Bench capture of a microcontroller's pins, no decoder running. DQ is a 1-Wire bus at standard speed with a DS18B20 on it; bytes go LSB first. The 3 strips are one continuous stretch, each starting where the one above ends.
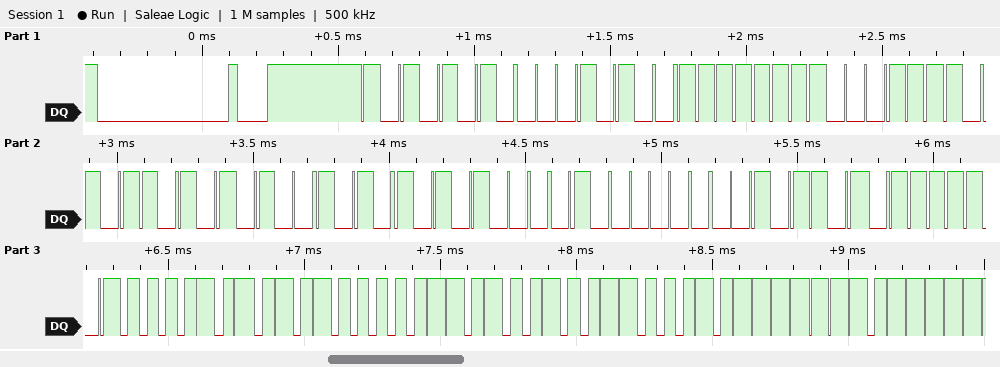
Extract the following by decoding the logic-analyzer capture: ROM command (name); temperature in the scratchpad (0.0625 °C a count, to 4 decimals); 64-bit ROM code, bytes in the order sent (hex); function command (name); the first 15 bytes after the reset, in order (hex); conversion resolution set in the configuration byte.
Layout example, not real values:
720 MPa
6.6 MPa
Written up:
Match ROM
85.0000 °C
28 FF 78 AD 52 15 02 B4
Read Scratchpad
55 28 FF 78 AD 52 15 02 B4 BE 50 05 4B 46 7F
12 bits
